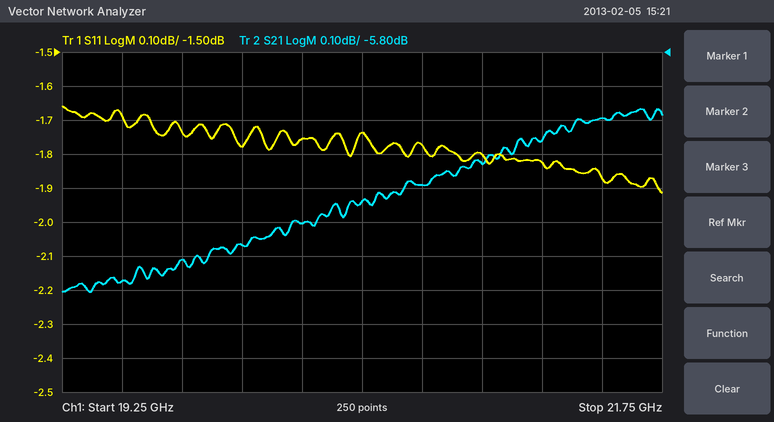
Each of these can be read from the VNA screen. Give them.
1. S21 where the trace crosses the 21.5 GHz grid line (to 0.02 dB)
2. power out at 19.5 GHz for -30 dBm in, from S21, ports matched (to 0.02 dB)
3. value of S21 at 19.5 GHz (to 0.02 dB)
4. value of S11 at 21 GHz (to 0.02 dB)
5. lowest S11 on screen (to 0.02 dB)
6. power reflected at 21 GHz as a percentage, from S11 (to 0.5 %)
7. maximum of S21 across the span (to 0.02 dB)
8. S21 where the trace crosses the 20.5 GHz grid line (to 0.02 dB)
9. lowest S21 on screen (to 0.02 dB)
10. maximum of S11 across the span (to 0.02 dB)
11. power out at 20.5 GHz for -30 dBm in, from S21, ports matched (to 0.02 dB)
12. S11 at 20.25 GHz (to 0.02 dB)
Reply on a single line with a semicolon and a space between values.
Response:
-6.00 dB; -36.48 dBm; -6.48 dB; -1.80 dB; -1.92 dB; 66.0 %; -5.96 dB; -6.24 dB; -6.50 dB; -1.66 dB; -36.24 dBm; -1.76 dB
